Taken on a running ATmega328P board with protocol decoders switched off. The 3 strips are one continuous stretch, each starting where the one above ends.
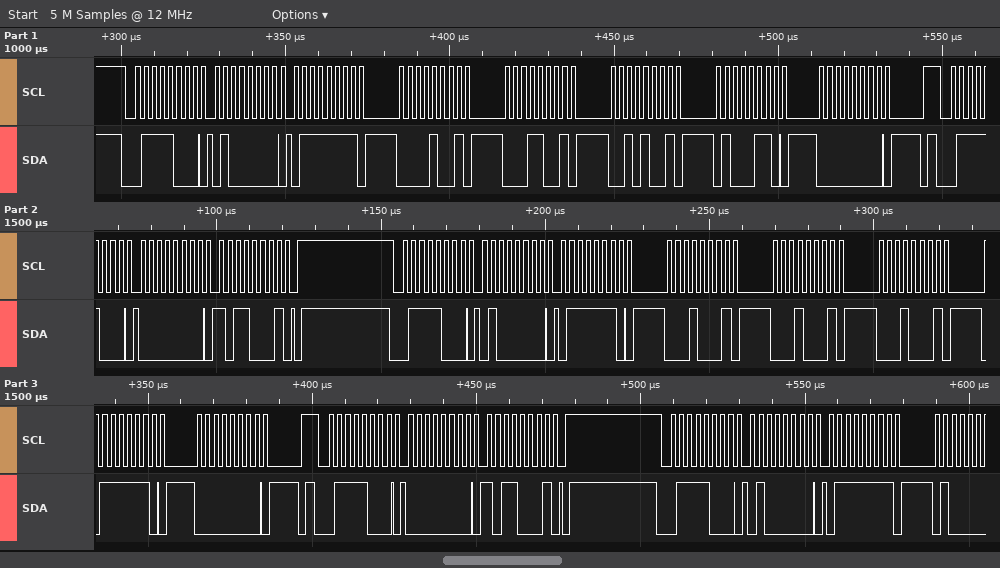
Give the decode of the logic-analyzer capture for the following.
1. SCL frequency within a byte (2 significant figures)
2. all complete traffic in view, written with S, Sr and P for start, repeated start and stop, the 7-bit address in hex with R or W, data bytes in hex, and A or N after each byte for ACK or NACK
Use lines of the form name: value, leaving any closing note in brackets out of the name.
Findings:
SCL frequency within a byte: 400 kHz
all complete traffic in view, written with S, Sr and P for start, repeated start and stop, the 7-bit address in hex with R or W, data bytes in hex, and A or N after each byte for ACK or NACK: S 3CW A 40 A 7F A 09 A 19 A 29 A 46 A 00 A P S 3CW A 00 A B1 A P S 3CW A 40 A 7E A 11 A 11 A 11 A 7E A 00 A P S 3CW A 00 A B1 A P S 3CW A 40 A 7F A
